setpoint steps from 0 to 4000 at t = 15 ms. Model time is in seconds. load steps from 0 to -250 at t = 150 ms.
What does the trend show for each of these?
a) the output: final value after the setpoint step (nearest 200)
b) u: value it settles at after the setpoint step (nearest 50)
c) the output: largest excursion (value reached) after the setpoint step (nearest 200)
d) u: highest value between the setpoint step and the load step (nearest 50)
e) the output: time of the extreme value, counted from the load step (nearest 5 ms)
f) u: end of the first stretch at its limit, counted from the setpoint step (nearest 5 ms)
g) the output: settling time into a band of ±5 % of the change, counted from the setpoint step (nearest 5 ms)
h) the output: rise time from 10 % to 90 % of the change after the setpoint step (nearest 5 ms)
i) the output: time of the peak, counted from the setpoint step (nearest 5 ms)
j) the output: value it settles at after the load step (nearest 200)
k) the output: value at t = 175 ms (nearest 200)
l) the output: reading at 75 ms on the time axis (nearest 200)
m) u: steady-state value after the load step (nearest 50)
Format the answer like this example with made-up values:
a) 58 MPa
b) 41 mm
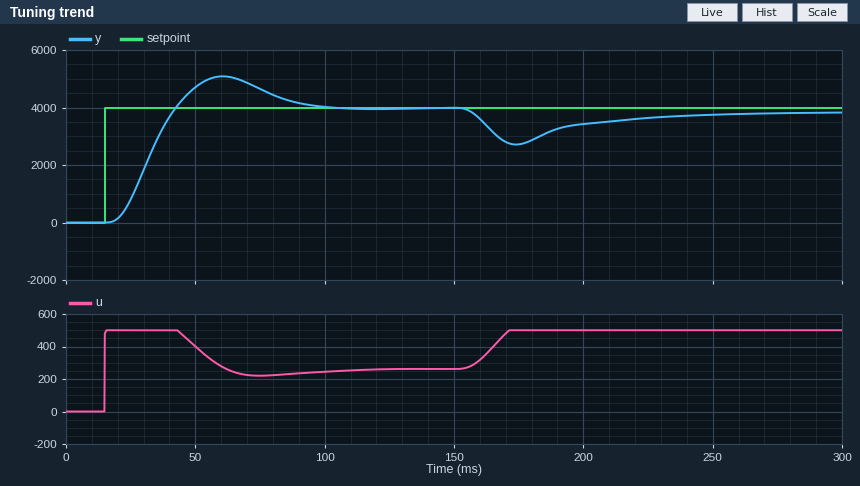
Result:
a) 4000
b) 250
c) 5000
d) 500
e) 25 ms
f) 30 ms
g) 75 ms
h) 15 ms
i) 45 ms
j) 3800
k) 2800
l) 4600
m) 500
